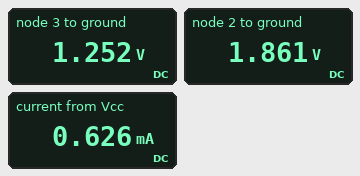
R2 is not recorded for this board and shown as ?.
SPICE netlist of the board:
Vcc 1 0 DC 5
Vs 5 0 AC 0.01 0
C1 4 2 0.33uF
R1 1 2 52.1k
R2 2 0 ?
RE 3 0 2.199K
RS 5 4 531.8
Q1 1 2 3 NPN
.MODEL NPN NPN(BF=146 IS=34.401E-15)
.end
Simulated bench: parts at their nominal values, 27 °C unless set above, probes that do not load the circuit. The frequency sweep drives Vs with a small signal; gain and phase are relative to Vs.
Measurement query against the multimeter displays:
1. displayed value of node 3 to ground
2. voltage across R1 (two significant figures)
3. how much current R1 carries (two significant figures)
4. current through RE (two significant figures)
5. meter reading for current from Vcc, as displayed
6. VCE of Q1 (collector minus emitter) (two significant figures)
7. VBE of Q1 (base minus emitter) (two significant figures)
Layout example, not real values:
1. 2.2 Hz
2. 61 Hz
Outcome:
1. 1.252 V
2. 3.1 V
3. 60 µA
4. 570 µA
5. 0.626 mA
6. 3.7 V
7. 610 mV
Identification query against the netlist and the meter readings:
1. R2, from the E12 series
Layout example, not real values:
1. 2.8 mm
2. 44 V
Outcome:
1. 33 kΩ
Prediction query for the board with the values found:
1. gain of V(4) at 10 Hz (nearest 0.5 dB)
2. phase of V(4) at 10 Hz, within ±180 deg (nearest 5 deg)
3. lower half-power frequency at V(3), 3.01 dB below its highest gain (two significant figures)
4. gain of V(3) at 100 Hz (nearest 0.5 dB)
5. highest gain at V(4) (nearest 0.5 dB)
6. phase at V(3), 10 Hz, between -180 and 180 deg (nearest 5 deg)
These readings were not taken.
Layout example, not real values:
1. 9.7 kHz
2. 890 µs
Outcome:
1. 0 dB
2. 0 deg
3. 25 Hz
4. -0.5 dB
5. 0 dB
6. 70 deg
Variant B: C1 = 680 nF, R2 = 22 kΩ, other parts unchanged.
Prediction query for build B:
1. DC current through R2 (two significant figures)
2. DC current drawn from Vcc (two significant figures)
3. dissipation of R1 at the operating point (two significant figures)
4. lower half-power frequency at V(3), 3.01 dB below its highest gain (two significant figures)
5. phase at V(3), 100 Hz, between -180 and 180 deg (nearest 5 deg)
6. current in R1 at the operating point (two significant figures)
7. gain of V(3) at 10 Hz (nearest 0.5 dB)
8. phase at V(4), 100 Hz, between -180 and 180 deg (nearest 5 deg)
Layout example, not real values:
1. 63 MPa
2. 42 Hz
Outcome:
1. 66 µA
2. 450 µA
3. 240 µW
4. 15 Hz
5. 10 deg
6. 68 µA
7. -6.0 dB
8. 0 deg
